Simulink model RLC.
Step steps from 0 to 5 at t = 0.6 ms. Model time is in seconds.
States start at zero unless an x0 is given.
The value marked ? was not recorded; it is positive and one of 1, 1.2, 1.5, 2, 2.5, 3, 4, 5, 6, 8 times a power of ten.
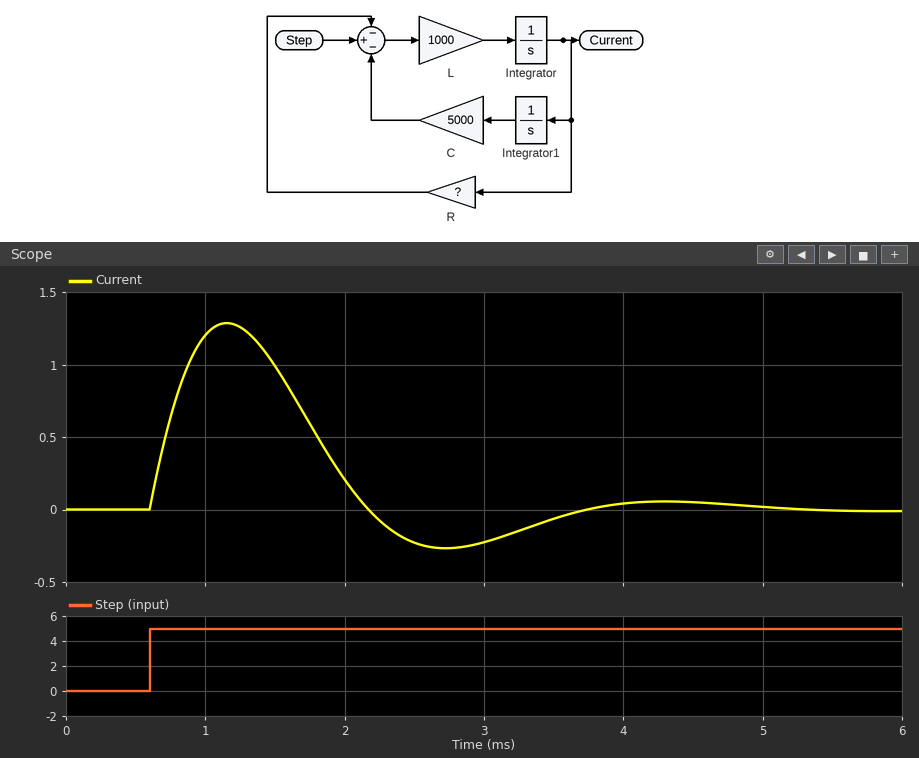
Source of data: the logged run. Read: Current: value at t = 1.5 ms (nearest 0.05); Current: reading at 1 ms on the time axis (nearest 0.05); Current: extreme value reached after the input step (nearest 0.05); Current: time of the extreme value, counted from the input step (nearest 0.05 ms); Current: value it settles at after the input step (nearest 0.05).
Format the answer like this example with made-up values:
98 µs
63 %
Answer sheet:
1.00
1.20
1.30
0.55 ms
0.00
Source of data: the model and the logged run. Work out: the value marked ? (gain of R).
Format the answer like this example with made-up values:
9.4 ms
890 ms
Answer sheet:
2
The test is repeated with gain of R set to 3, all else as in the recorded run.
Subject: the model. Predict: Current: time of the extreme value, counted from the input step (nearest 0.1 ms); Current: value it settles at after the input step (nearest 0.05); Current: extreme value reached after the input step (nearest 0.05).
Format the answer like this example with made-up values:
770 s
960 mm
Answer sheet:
0.5 ms
0.00
1.05
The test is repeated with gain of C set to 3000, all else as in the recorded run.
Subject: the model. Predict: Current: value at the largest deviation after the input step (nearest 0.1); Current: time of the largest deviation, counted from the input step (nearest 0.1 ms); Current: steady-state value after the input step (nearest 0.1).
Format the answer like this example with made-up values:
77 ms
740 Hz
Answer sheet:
1.5
0.7 ms
0.0
